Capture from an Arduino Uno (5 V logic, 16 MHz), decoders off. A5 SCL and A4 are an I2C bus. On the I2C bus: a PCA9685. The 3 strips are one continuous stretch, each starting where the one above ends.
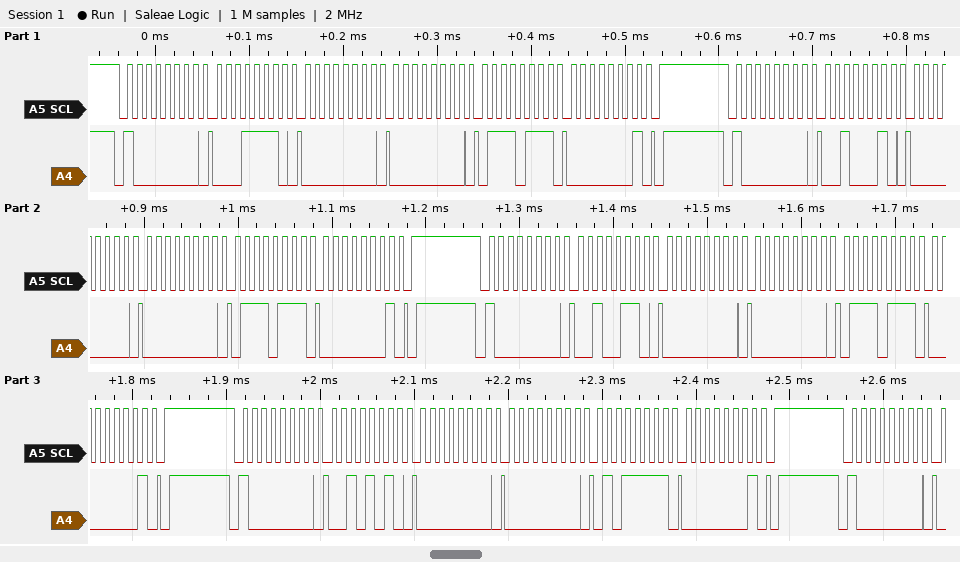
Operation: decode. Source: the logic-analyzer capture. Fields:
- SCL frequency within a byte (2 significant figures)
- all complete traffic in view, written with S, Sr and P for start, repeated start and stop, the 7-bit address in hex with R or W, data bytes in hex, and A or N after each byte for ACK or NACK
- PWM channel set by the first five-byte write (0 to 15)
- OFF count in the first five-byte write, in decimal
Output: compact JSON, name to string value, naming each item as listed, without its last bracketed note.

{"SCL frequency within a byte": "100 kHz", "all complete traffic in view, written with S, Sr and P for start, repeated start and stop, the 7-bit address in hex with R or W, data bytes in hex, and A or N after each byte for ACK or NACK": "S 40W A 1E A 00 A 00 A 77 A 01 A P S 40W A 22 A 00 A 00 A 77 A 01 A P S 40W A 26 A 00 A 00 A 77 A 01 A P S 40W A 2A A 00 A 00 A 5F A 01 A P S 40W A", "PWM channel set by the first five-byte write": "6", "OFF count in the first five-byte write, in decimal": "375"}
